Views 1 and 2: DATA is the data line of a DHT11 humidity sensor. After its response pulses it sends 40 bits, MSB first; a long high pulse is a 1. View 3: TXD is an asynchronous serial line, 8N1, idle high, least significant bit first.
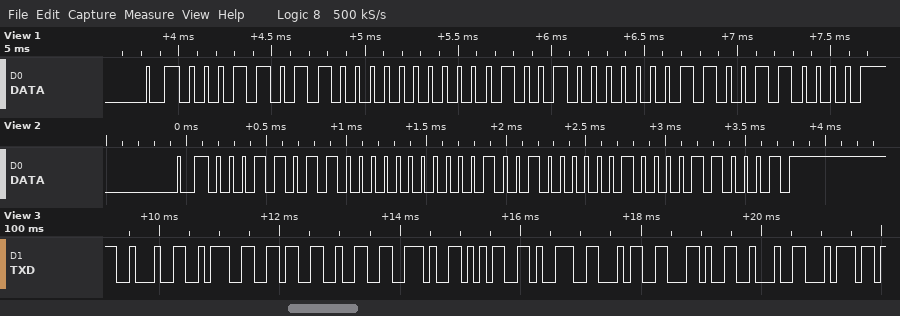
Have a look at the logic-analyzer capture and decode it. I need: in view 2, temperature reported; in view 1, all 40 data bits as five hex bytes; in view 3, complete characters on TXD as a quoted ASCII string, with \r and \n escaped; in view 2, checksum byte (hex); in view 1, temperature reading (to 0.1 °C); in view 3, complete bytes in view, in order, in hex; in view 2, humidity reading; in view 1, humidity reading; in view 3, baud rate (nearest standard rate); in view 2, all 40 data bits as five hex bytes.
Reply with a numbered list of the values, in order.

1. 18.4 °C
2. 1B 00 12 03 30
3. "\":62.594,\"t"
4. 0x31
5. 18.3 °C
6. 22 3A 36 32 2E 35 39 34 2C 22 74
7. 27 %
8. 27 %
9. 9600 baud
10. 1B 00 12 04 31
